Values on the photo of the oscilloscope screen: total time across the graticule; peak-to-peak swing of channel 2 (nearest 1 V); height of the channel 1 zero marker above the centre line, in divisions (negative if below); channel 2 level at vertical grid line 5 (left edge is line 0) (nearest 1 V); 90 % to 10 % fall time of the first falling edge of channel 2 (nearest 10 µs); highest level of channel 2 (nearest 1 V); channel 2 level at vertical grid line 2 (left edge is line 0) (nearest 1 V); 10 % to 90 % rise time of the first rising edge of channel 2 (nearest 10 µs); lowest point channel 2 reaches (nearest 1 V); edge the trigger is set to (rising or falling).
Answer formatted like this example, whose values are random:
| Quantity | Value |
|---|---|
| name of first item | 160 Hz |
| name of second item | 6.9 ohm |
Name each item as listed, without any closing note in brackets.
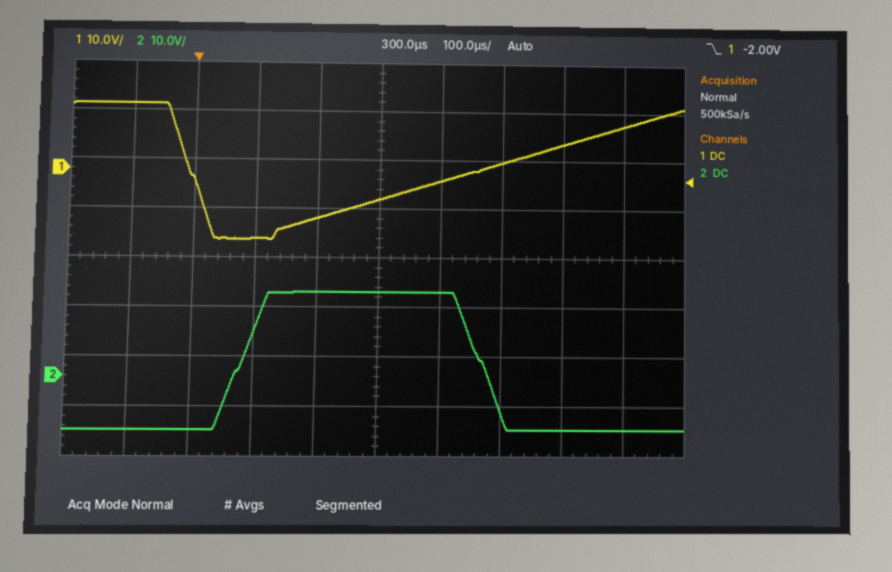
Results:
| Quantity | Value |
|---|---|
| total time across the graticule | 1 ms |
| peak-to-peak swing of channel 2 | 28 V |
| height of the channel 1 zero marker above the centre line, in divisions | +1.8 div |
| channel 2 level at vertical grid line 5 (left edge is line 0) | 17 V |
| 90 % to 10 % fall time of the first falling edge of channel 2 | 70 µs |
| highest level of channel 2 | 17 V |
| channel 2 level at vertical grid line 2 (left edge is line 0) | -11 V |
| 10 % to 90 % rise time of the first rising edge of channel 2 | 70 µs |
| lowest point channel 2 reaches | -11 V |
| edge the trigger is set to | falling |
